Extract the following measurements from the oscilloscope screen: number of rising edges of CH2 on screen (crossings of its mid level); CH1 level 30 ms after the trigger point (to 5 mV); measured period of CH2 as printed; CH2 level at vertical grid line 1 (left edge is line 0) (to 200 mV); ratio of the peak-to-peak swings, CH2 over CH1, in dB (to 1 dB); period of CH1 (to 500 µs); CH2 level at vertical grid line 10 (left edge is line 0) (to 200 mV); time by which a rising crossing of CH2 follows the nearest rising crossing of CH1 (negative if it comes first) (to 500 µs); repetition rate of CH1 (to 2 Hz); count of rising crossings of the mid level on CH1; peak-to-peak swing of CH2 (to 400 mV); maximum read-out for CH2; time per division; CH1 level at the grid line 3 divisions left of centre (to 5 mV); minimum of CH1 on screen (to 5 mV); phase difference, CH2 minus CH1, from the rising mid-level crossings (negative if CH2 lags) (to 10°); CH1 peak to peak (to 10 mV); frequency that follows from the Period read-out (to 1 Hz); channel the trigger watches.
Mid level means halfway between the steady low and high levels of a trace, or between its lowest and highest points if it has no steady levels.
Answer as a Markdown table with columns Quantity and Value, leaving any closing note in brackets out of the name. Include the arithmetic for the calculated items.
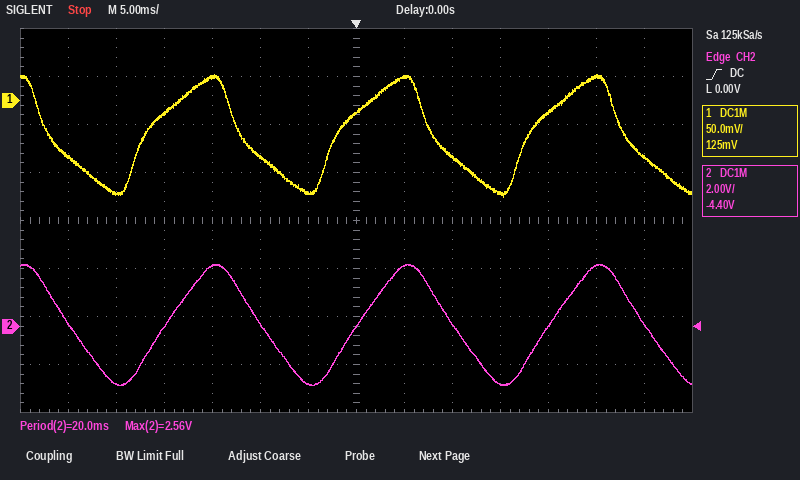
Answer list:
| Quantity | Value |
|---|---|
| number of rising edges of CH2 on screen | 3 |
| CH1 level 30 ms after the trigger point | -60 mV |
| measured period of CH2 as printed | 20.0 ms |
| CH2 level at vertical grid line 1 (left edge is line 0) | 200 mV |
| ratio of the peak-to-peak swings, CH2 over CH1, in dB | 20 log10(5.2 V / 130 mV) ≈ 32 dB |
| period of CH1 | 20.0 ms |
| CH2 level at vertical grid line 10 (left edge is line 0) | -2.4 V |
| time by which a rising crossing of CH2 follows the nearest rising crossing of CH1 (negative if it comes first) | +2.0 ms |
| repetition rate of CH1 | 1 / 20.0 ms ≈ 50 Hz |
| count of rising crossings of the mid level on CH1 | 3 |
| peak-to-peak swing of CH2 | 5.2 V |
| maximum read-out for CH2 | 2.56 V |
| time per division | 5 ms |
| CH1 level at the grid line 3 divisions left of centre | 25 mV |
| minimum of CH1 on screen | -100 mV |
| phase difference, CH2 minus CH1, from the rising mid-level crossings (negative if CH2 lags) | −360° × (+2.0 ms) / 20.0 ms ≈ -36.0°, so -40° to the nearest 10° |
| CH1 peak to peak | 130 mV |
| frequency that follows from the Period read-out | 1 / 20.0 ms ≈ 50 Hz |
| channel the trigger watches | CH2 |
